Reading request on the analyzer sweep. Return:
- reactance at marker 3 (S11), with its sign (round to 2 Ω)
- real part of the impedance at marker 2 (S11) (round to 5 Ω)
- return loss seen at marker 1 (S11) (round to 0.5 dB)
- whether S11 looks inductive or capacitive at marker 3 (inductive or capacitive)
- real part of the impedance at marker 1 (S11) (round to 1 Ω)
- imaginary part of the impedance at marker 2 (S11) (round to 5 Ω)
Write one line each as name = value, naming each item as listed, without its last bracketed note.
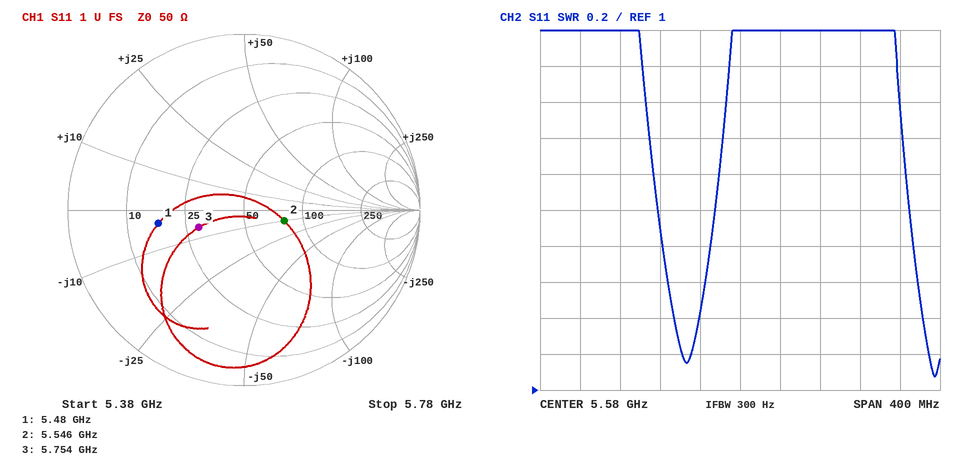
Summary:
reactance at marker 3 (S11), with its sign = -6 Ω
real part of the impedance at marker 2 (S11) = 80 Ω
return loss seen at marker 1 (S11) = 6.0 dB
whether S11 looks inductive or capacitive at marker 3 = capacitive
real part of the impedance at marker 1 (S11) = 17 Ω
imaginary part of the impedance at marker 2 (S11) = -10 Ω
